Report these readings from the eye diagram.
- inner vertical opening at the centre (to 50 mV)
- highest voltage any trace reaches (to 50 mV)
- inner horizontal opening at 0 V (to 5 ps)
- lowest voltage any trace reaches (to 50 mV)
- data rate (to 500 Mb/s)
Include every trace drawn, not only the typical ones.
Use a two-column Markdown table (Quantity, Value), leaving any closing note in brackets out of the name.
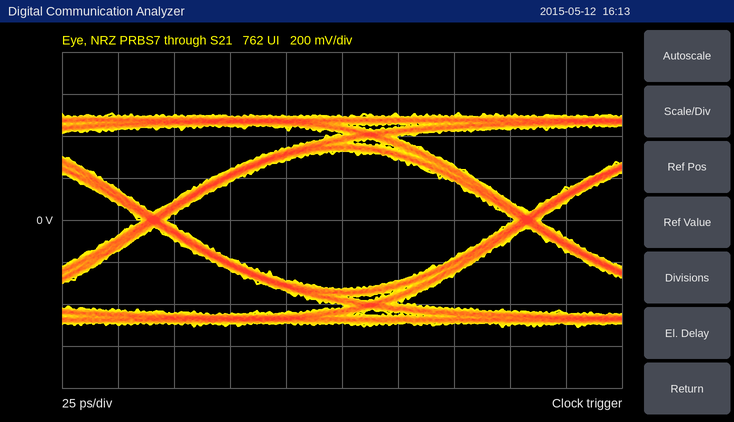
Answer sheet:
| Quantity | Value |
|---|---|
| inner vertical opening at the centre | 650 mV |
| highest voltage any trace reaches | 500 mV |
| inner horizontal opening at 0 V | 155 ps |
| lowest voltage any trace reaches | -500 mV |
| data rate | 6.0 Gb/s |
